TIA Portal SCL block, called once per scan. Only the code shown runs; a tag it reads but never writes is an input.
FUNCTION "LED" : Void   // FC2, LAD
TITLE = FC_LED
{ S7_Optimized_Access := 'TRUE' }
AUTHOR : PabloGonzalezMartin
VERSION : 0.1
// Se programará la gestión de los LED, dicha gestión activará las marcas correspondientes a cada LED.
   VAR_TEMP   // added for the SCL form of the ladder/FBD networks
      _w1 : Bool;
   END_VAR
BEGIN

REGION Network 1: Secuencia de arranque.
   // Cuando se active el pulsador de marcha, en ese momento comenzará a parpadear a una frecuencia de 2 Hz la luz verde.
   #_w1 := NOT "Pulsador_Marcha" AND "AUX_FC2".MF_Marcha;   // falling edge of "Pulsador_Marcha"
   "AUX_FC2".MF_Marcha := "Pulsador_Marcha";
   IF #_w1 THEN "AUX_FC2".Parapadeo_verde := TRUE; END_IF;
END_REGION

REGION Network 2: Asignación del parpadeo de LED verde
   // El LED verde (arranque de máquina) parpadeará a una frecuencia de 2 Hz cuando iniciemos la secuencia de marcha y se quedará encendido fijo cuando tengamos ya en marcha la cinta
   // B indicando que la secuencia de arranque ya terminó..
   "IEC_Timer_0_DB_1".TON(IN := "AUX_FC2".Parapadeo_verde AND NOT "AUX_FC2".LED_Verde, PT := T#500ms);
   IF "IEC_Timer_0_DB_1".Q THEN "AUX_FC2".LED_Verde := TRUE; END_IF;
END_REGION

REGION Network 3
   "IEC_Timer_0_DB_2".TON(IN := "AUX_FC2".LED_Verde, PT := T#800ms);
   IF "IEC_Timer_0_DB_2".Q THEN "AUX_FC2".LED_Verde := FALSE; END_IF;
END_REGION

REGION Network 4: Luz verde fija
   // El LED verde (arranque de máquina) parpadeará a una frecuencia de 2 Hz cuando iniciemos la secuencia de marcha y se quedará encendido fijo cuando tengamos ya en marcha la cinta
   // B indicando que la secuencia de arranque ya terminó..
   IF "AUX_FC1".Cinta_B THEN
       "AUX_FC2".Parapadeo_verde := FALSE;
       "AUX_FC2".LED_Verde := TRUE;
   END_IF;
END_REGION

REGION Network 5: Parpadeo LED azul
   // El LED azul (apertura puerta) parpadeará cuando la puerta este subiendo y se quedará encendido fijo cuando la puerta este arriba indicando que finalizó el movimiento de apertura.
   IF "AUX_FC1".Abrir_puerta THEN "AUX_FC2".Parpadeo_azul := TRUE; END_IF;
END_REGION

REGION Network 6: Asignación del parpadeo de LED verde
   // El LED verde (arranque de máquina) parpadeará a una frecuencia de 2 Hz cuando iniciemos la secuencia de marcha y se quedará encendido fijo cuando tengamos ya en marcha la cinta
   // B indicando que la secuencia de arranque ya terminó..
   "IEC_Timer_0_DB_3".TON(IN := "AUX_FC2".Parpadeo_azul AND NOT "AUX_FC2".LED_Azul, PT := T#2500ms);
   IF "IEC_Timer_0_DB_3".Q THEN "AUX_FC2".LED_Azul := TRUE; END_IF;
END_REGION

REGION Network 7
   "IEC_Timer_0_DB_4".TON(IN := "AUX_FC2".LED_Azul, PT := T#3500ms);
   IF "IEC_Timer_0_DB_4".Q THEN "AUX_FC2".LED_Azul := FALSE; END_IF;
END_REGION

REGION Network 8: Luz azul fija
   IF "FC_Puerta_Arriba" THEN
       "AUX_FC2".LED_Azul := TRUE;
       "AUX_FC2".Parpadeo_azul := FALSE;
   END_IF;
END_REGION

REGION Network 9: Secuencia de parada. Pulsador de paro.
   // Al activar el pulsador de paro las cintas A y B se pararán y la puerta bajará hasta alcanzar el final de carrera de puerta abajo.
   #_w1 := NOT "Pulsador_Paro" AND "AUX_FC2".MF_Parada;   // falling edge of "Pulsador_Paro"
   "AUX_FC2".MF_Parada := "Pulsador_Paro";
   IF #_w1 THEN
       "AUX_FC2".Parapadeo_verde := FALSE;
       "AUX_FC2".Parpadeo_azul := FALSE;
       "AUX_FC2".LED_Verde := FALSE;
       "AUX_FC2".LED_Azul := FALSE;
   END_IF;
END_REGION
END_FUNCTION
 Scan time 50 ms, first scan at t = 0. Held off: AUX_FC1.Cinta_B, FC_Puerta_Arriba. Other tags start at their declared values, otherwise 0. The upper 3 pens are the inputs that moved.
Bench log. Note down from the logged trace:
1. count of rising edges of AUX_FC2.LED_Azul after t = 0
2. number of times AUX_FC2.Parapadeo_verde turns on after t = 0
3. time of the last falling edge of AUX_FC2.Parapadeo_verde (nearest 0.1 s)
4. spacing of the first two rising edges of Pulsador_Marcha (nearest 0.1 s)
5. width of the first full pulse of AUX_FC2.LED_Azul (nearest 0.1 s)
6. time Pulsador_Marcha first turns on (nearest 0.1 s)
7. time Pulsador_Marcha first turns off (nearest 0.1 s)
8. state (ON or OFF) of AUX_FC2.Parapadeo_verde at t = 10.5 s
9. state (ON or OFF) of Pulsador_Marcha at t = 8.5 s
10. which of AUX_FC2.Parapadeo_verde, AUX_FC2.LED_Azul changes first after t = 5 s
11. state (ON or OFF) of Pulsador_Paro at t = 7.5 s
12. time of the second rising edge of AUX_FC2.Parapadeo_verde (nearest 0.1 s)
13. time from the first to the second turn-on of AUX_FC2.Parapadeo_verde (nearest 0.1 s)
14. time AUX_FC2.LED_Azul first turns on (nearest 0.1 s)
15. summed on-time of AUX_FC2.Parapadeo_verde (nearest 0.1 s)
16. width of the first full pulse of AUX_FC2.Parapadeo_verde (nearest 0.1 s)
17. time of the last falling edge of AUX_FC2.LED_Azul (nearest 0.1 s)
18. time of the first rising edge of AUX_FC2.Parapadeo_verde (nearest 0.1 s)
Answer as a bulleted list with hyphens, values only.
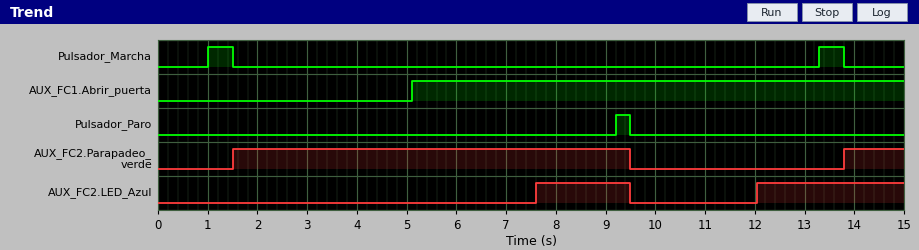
- 2
- 2
- 9.5 s
- 12.3 s
- 1.9 s
- 1.0 s
- 1.5 s
- OFF
- OFF
- AUX_FC2.LED_Azul
- OFF
- 13.8 s
- 12.3 s
- 7.6 s
- 9.2 s
- 8.0 s
- 9.5 s
- 1.5 s
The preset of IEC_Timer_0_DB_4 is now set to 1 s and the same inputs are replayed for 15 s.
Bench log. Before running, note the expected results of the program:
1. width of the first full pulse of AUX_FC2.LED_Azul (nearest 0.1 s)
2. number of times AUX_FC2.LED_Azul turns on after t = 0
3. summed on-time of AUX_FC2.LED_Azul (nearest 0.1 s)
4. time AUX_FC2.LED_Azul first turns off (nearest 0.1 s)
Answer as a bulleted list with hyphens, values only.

- 1.0 s
- 3
- 2.3 s
- 8.6 s
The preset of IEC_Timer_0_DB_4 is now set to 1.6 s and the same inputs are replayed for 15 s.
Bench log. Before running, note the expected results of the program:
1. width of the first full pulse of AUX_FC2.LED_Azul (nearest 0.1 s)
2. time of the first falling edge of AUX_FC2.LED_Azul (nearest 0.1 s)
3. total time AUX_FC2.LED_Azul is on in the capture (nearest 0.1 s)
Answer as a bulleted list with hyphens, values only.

- 1.6 s
- 9.2 s
- 3.2 s
